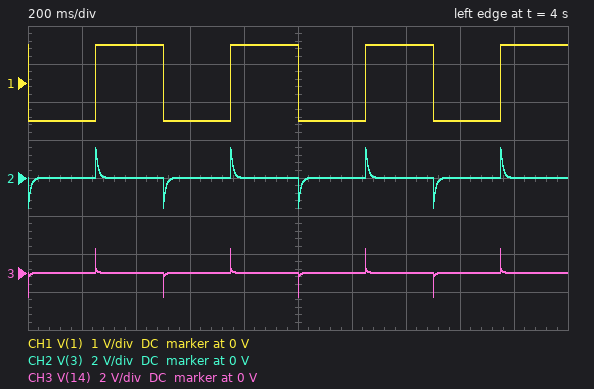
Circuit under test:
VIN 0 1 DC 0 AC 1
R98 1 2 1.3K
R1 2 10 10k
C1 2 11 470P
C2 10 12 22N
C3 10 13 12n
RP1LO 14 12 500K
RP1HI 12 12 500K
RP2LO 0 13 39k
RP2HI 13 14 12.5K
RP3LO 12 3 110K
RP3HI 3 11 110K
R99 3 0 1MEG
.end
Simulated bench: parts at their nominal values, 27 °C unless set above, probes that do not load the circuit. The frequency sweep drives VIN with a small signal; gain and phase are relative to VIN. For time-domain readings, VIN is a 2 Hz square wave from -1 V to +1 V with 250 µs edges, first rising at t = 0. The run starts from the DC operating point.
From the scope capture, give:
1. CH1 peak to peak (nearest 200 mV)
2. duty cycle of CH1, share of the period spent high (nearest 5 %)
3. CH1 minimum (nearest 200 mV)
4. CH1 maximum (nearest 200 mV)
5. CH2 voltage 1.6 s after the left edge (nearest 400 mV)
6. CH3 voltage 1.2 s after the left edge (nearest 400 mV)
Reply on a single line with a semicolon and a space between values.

2.0 V; 50 %; -1.0 V; 1.0 V; 0 V; 0 V
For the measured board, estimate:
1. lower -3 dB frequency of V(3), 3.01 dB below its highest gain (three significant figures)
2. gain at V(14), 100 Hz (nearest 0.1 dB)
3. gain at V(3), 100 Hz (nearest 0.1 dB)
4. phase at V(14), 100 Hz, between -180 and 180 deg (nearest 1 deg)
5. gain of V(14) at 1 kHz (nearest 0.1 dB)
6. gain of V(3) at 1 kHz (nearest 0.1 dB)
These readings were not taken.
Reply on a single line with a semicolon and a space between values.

17.3 Hz; -11.1 dB; -1.2 dB; -127 deg; -2.6 dB; -2.6 dB
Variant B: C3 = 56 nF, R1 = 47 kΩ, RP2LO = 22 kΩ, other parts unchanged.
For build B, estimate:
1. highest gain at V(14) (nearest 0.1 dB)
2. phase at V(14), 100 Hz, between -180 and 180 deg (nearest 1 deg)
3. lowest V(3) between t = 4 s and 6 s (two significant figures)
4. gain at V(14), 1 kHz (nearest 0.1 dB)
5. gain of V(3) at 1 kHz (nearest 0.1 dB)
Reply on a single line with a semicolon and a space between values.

-9.1 dB; -159 deg; -980 mV; -9.9 dB; -7.7 dB
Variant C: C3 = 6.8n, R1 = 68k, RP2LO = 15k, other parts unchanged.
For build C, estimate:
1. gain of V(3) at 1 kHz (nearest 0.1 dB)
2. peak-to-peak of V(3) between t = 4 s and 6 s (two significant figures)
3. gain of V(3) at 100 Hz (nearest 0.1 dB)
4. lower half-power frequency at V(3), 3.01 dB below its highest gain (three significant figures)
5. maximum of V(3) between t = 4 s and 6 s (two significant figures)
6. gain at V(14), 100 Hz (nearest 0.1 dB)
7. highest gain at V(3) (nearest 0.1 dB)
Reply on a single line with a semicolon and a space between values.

-9.8 dB; 2.6 V; -2.9 dB; 15.0 Hz; 1.3 V; -23.0 dB; -2.8 dB
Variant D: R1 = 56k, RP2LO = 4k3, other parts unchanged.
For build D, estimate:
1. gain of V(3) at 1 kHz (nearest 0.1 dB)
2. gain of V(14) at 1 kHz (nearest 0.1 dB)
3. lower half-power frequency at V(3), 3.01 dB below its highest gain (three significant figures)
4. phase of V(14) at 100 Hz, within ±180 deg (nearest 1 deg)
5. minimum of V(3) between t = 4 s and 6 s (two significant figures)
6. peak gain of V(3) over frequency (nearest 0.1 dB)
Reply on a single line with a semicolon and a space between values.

-13.2 dB; -23.0 dB; 15.1 Hz; -152 deg; -1.3 V; -2.8 dB
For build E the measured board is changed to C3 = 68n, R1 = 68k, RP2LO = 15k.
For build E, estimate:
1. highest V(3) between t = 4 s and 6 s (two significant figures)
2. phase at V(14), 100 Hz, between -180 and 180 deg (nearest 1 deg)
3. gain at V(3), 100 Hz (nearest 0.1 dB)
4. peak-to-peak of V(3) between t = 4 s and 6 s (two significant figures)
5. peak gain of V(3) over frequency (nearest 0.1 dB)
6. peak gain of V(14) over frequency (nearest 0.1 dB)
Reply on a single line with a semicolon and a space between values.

800 mV; -165 deg; -10.8 dB; 1.6 V; -4.9 dB; -13.3 dB
